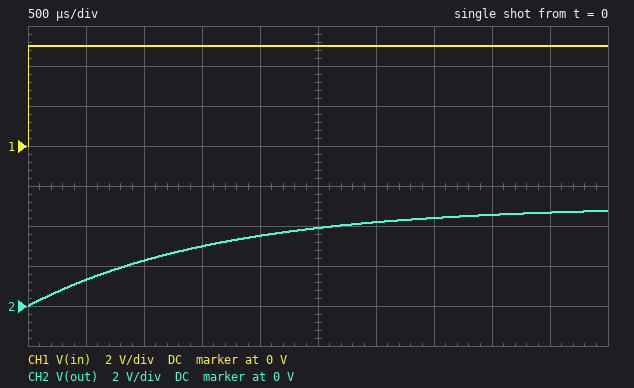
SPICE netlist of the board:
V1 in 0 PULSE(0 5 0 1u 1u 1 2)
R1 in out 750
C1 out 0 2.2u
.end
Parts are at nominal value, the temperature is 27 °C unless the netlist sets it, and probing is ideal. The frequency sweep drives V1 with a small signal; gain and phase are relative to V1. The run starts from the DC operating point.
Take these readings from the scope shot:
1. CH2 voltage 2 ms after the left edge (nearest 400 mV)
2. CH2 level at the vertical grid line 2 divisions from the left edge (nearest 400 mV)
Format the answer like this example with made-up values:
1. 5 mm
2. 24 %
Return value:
1. 3.6 V
2. 2.4 V
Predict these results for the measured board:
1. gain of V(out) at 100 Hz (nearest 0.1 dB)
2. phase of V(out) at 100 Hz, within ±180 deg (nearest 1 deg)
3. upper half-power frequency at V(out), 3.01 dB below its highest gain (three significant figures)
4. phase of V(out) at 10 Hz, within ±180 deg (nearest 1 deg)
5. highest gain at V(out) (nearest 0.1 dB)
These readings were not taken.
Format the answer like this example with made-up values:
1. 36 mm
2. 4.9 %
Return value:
1. -3.2 dB
2. -46 deg
3. 96.5 Hz
4. -6 deg
5. 0 dB
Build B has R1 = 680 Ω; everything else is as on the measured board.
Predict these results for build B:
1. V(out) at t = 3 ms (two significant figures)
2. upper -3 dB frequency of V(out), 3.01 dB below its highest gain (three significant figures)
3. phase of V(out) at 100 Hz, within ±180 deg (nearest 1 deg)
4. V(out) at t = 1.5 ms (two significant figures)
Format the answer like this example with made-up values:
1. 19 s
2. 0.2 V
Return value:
1. 4.3 V
2. 106 Hz
3. -43 deg
4. 3.2 V
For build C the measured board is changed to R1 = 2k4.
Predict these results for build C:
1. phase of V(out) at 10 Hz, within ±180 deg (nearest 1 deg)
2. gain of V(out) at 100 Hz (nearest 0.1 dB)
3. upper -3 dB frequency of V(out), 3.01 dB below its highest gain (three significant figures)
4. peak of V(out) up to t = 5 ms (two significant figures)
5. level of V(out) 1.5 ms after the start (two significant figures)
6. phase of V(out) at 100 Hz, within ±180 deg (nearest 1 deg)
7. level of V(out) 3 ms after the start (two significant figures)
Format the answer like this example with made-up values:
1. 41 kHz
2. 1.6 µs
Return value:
1. -18 deg
2. -10.8 dB
3. 30.1 Hz
4. 3.1 V
5. 1.2 V
6. -73 deg
7. 2.2 V
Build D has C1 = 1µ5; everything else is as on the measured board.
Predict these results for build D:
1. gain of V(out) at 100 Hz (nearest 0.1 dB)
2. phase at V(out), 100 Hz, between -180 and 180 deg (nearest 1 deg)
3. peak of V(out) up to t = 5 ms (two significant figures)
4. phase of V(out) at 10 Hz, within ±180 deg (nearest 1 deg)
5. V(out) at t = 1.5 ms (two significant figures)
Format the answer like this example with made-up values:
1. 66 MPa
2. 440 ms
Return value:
1. -1.8 dB
2. -35 deg
3. 4.9 V
4. -4 deg
5. 3.7 V
